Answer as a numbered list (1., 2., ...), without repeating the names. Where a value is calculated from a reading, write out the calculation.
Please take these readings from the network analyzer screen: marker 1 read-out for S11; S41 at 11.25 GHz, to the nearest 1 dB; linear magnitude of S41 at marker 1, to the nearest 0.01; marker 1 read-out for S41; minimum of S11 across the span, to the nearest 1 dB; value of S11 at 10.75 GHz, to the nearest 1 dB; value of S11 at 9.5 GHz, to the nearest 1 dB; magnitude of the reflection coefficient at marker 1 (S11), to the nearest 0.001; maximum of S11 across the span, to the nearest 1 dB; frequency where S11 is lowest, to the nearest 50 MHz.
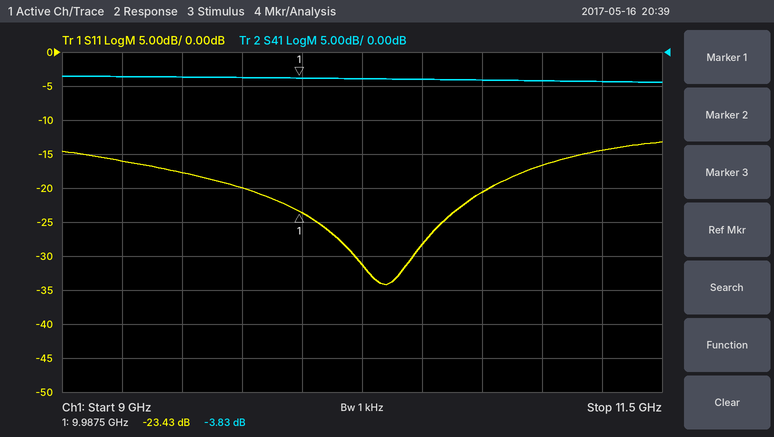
1. -23.43 dB
2. -4 dB
3. 10^(-3.83/20) ≈ 0.64
4. -3.83 dB
5. -34 dB
6. -21 dB
7. -18 dB
8. 10^(-23.43/20) ≈ 0.067
9. -13 dB
10. 10.35 GHz
